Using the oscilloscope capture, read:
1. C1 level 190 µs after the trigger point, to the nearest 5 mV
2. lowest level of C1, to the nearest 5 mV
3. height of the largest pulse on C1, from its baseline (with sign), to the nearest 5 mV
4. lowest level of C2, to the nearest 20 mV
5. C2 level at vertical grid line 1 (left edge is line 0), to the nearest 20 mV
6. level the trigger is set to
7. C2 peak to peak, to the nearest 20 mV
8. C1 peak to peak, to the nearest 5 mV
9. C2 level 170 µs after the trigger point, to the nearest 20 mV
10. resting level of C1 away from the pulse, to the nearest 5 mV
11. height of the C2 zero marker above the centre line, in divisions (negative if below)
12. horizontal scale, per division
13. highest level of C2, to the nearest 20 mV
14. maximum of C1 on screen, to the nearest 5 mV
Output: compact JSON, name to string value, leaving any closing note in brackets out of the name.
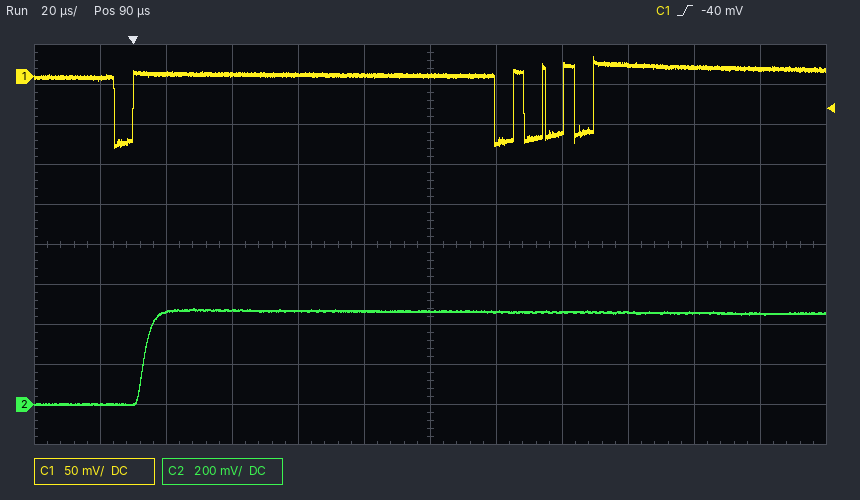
{"C1 level 190 µs after the trigger point, to the nearest 5 mV": "10 mV", "lowest level of C1, to the nearest 5 mV": "-90 mV", "height of the largest pulse on C1, from its baseline (with sign), to the nearest 5 mV": "-90 mV", "lowest level of C2, to the nearest 20 mV": "0 mV", "C2 level at vertical grid line 1 (left edge is line 0), to the nearest 20 mV": "0 mV", "level the trigger is set to": "-40 mV", "C2 peak to peak, to the nearest 20 mV": "480 mV", "C1 peak to peak, to the nearest 5 mV": "115 mV", "C2 level 170 µs after the trigger point, to the nearest 20 mV": "460 mV", "resting level of C1 away from the pulse, to the nearest 5 mV": "0 mV", "height of the C2 zero marker above the centre line, in divisions": "-4.0 div", "horizontal scale, per division": "20 µs", "highest level of C2, to the nearest 20 mV": "480 mV", "maximum of C1 on screen, to the nearest 5 mV": "25 mV"}
